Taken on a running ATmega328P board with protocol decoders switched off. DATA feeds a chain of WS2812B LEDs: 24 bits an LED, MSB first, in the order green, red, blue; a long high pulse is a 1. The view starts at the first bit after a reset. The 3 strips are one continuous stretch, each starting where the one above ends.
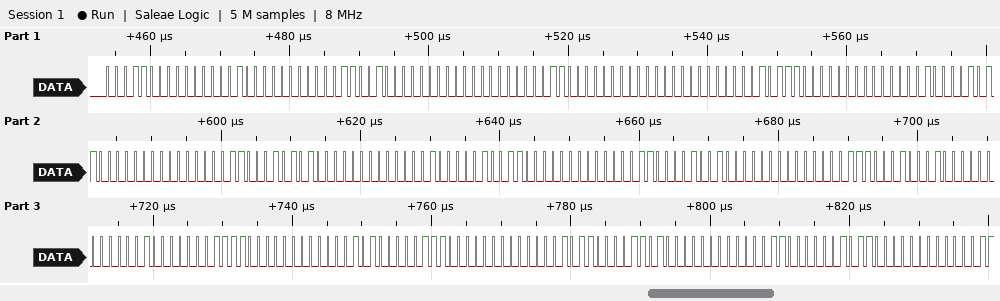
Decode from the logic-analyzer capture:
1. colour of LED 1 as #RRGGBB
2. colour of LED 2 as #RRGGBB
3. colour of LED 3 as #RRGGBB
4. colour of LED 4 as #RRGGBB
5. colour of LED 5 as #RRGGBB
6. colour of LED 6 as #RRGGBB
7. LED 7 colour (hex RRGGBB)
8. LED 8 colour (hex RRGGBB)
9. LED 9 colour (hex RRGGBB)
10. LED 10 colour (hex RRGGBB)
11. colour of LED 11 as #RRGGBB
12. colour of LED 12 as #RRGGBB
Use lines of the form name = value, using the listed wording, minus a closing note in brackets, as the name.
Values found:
colour of LED 1 as #RRGGBB = #011800
colour of LED 2 as #RRGGBB = #001900
colour of LED 3 as #RRGGBB = #001800
colour of LED 4 as #RRGGBB = #001702
colour of LED 5 as #RRGGBB = #001603
colour of LED 6 as #RRGGBB = #001504
LED 7 colour = #001306
LED 8 colour = #001207
LED 9 colour = #001108
LED 10 colour = #000F0A
colour of LED 11 as #RRGGBB = #000E0B
colour of LED 12 as #RRGGBB = #000D0C
